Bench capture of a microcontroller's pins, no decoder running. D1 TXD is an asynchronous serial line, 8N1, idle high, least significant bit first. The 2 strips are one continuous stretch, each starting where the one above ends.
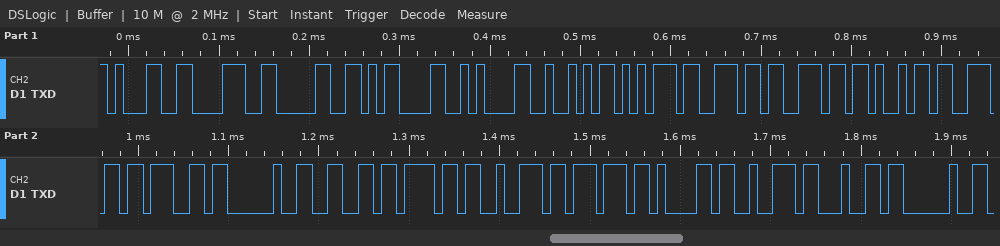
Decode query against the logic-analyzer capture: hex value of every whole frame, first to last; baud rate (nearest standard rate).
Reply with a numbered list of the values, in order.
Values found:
1. 31 38 30 0D 0A 52 75 6E 6E 69 6E 67 20 66 6F 72 77 61 72 64 20
2. 115200 baud
